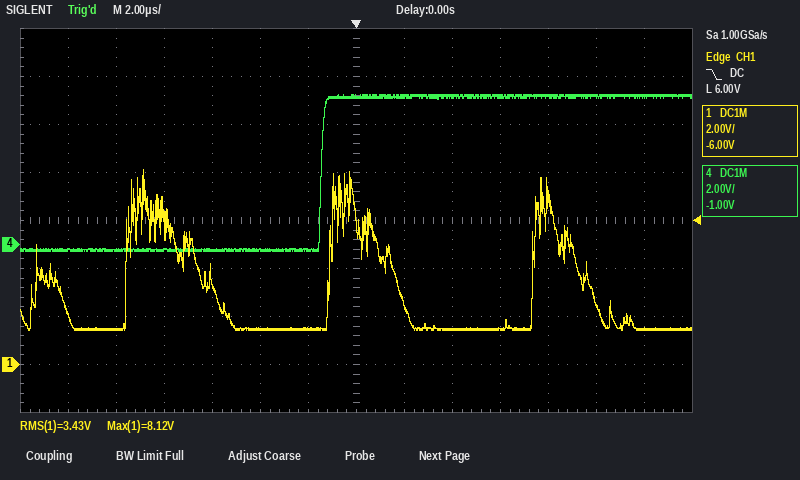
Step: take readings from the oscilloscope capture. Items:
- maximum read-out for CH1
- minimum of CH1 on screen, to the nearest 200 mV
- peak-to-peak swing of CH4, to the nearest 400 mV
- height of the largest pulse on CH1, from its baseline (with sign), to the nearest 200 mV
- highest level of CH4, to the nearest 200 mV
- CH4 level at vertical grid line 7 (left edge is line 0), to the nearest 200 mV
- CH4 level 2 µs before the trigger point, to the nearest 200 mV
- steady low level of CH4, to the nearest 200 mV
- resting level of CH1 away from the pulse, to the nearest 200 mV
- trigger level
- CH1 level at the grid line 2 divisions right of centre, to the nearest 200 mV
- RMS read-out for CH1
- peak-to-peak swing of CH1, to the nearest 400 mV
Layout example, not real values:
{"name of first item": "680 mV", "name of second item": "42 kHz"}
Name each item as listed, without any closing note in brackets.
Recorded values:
{"maximum read-out for CH1": "8.12 V", "minimum of CH1 on screen, to the nearest 200 mV": "1.4 V", "peak-to-peak swing of CH4, to the nearest 400 mV": "6.4 V", "height of the largest pulse on CH1, from its baseline (with sign), to the nearest 200 mV": "+6.6 V", "highest level of CH4, to the nearest 200 mV": "6.2 V", "CH4 level at vertical grid line 7 (left edge is line 0), to the nearest 200 mV": "6.2 V", "CH4 level 2 µs before the trigger point, to the nearest 200 mV": "-200 mV", "steady low level of CH4, to the nearest 200 mV": "-200 mV", "resting level of CH1 away from the pulse, to the nearest 200 mV": "1.4 V", "trigger level": "6.00 V", "CH1 level at the grid line 2 divisions right of centre, to the nearest 200 mV": "1.4 V", "RMS read-out for CH1": "3.43 V", "peak-to-peak swing of CH1, to the nearest 400 mV": "6.8 V"}
